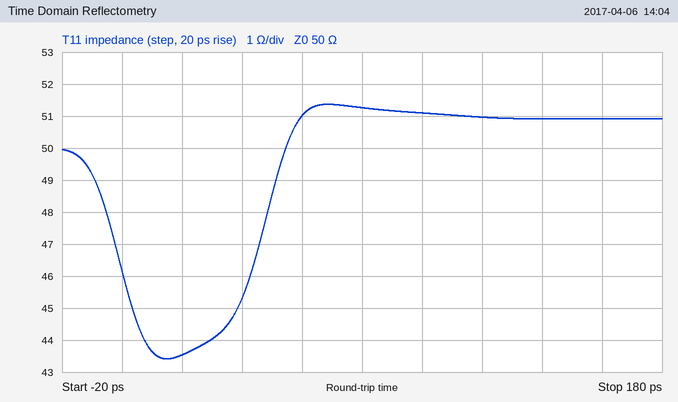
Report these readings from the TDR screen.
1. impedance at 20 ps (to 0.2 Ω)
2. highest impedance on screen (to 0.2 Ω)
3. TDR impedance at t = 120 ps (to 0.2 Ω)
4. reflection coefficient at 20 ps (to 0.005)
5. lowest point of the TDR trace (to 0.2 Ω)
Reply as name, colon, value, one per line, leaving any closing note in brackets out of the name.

impedance at 20 ps: 43.6 Ω
highest impedance on screen: 51.4 Ω
TDR impedance at t = 120 ps: 51.0 Ω
reflection coefficient at 20 ps: -0.070
lowest point of the TDR trace: 43.4 Ω
